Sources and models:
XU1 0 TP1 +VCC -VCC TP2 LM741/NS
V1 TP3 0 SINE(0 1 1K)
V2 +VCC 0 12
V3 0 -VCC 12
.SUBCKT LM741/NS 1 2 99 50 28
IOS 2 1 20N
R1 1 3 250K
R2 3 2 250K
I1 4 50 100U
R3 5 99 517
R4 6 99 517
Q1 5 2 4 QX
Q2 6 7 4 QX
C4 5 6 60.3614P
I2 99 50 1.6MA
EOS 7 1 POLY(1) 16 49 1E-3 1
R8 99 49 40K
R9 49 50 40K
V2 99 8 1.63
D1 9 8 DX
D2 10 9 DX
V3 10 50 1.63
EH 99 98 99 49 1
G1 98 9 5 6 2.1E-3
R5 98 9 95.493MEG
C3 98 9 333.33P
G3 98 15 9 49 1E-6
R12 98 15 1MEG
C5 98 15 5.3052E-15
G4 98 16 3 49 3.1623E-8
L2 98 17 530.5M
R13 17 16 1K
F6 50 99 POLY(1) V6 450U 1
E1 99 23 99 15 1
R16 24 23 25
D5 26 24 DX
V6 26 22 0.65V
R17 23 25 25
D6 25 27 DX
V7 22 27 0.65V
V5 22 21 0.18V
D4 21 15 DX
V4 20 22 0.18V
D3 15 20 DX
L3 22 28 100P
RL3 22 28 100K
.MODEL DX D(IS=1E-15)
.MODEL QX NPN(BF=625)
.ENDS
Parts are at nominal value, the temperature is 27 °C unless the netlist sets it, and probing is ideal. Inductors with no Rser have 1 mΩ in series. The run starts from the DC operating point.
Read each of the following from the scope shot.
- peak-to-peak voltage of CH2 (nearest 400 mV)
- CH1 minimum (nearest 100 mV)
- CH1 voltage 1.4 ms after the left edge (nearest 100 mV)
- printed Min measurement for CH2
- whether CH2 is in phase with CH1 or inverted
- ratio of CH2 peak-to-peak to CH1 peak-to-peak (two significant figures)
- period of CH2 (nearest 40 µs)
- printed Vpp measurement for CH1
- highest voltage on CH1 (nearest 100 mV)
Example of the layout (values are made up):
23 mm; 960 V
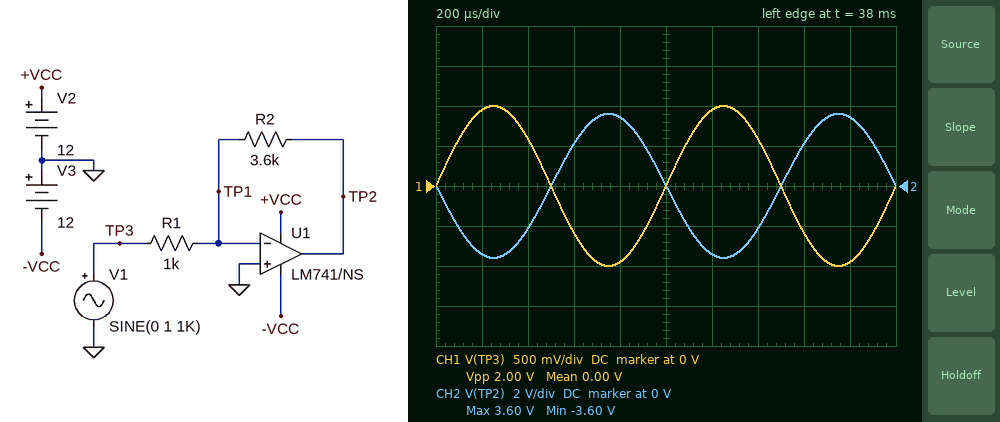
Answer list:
7.2 V; -1.0 V; 600 mV; -3.60 V; inverted; 3.6; 1.00 ms; 2.00 V; 1.0 V
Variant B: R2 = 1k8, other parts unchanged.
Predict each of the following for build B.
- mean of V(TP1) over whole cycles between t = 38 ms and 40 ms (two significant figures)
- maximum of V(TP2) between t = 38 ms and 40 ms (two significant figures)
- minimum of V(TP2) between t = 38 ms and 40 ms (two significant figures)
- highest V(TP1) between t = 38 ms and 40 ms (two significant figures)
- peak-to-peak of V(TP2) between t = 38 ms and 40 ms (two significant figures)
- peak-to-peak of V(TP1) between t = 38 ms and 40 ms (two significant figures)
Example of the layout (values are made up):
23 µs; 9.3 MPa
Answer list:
1.0 mV; 1.8 V; -1.8 V; 3.0 mV; 3.6 V; 4.0 mV
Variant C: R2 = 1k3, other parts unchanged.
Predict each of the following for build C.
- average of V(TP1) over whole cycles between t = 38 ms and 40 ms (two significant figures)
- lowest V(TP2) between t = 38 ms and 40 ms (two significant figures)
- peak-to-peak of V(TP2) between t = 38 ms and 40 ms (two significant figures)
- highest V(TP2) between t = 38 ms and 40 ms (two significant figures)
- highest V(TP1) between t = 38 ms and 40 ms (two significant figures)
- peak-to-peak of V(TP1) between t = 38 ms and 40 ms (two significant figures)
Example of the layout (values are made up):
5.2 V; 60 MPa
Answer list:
1.0 mV; -1.3 V; 2.6 V; 1.3 V; 2.5 mV; 3.0 mV
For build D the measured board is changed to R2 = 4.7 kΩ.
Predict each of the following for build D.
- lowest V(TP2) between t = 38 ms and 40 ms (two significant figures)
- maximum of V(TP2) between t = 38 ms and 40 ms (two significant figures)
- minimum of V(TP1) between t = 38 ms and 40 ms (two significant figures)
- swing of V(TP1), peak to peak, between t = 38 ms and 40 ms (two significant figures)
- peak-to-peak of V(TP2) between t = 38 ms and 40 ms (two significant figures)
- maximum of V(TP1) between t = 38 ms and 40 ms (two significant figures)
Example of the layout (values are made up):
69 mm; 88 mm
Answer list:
-4.7 V; 4.7 V; -3.9 mV; 9.8 mV; 9.4 V; 5.9 mV
